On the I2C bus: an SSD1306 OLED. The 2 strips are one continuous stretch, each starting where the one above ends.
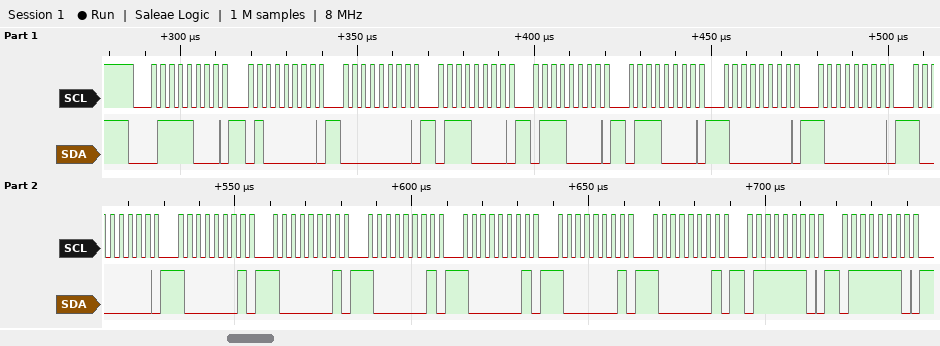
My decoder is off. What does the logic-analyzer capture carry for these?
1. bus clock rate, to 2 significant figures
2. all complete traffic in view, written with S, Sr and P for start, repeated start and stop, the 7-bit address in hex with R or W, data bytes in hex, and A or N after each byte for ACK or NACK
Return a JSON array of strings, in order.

["400 kHz", "S 3CW A 40 A 00 A 70 A 70 A 70 A 80 A 80 A 80 A 81 A 81 A 81 A 81 A 81 A 81 A 7E A 7E A"]
